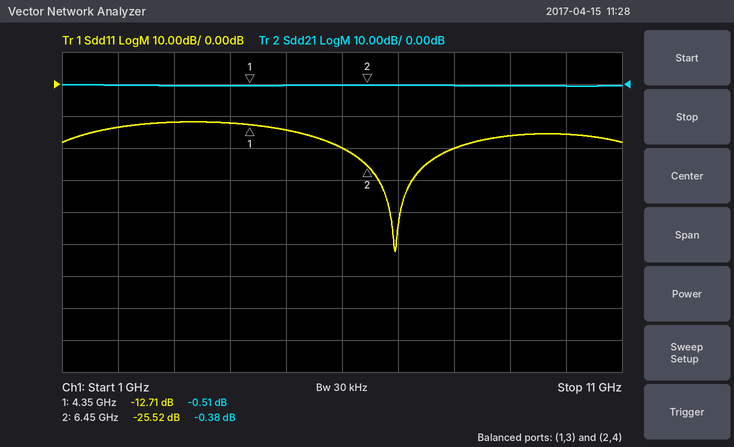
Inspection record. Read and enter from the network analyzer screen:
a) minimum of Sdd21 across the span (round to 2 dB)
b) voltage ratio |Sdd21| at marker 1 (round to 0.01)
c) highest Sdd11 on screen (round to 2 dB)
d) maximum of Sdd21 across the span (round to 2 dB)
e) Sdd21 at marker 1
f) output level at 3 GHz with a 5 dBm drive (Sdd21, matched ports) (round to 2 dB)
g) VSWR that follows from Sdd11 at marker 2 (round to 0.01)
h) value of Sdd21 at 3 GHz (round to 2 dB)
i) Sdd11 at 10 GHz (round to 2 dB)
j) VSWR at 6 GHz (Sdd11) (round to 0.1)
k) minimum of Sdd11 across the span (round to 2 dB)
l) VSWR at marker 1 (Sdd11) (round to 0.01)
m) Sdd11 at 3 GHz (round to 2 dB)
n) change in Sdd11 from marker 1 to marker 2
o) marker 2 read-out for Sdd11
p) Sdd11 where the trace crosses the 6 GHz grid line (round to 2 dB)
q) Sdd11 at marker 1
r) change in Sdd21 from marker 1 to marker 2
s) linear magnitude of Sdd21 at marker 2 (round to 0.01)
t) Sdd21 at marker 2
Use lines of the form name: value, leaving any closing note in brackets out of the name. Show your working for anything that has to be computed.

minimum of Sdd21 across the span: 0 dB
voltage ratio |Sdd21| at marker 1: 10^(-0.51/20) ≈ 0.94
highest Sdd11 on screen: -12 dB
maximum of Sdd21 across the span: 0 dB
Sdd21 at marker 1: -0.51 dB
output level at 3 GHz with a 5 dBm drive (Sdd21, matched ports): 5 dBm + (0 dB) = 4 dBm
VSWR that follows from Sdd11 at marker 2: (1 + 0.0530)/(1 − 0.0530) ≈ 1.11
value of Sdd21 at 3 GHz: 0 dB
Sdd11 at 10 GHz: -16 dB
VSWR at 6 GHz (Sdd11): |Γ| = 10^(-20/20) = 0.1000; VSWR = (1 + 0.1000)/(1 − 0.1000) ≈ 1.2
minimum of Sdd11 across the span: -52 dB
VSWR at marker 1 (Sdd11): (1 + 0.2315)/(1 − 0.2315) ≈ 1.60
Sdd11 at 3 GHz: -12 dB
change in Sdd11 from marker 1 to marker 2: -25.52 − (-12.71) = -12.81 dB
marker 2 read-out for Sdd11: -25.52 dB
Sdd11 where the trace crosses the 6 GHz grid line: -20 dB
Sdd11 at marker 1: -12.71 dB
change in Sdd21 from marker 1 to marker 2: -0.38 − (-0.51) = 0.13 dB
linear magnitude of Sdd21 at marker 2: 10^(-0.38/20) ≈ 0.96
Sdd21 at marker 2: -0.38 dB
